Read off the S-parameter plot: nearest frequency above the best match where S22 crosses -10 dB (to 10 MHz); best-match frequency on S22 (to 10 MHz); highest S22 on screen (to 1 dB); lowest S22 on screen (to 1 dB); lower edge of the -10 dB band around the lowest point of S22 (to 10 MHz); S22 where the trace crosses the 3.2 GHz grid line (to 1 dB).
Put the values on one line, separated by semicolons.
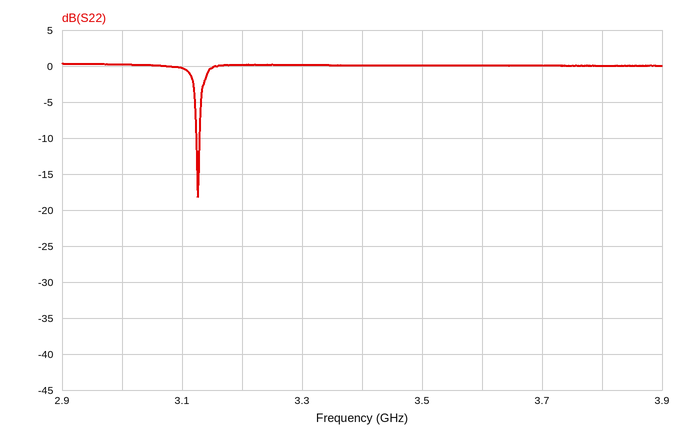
3.13 GHz; 3.13 GHz; 0 dB; -18 dB; 3.12 GHz; 0 dB
